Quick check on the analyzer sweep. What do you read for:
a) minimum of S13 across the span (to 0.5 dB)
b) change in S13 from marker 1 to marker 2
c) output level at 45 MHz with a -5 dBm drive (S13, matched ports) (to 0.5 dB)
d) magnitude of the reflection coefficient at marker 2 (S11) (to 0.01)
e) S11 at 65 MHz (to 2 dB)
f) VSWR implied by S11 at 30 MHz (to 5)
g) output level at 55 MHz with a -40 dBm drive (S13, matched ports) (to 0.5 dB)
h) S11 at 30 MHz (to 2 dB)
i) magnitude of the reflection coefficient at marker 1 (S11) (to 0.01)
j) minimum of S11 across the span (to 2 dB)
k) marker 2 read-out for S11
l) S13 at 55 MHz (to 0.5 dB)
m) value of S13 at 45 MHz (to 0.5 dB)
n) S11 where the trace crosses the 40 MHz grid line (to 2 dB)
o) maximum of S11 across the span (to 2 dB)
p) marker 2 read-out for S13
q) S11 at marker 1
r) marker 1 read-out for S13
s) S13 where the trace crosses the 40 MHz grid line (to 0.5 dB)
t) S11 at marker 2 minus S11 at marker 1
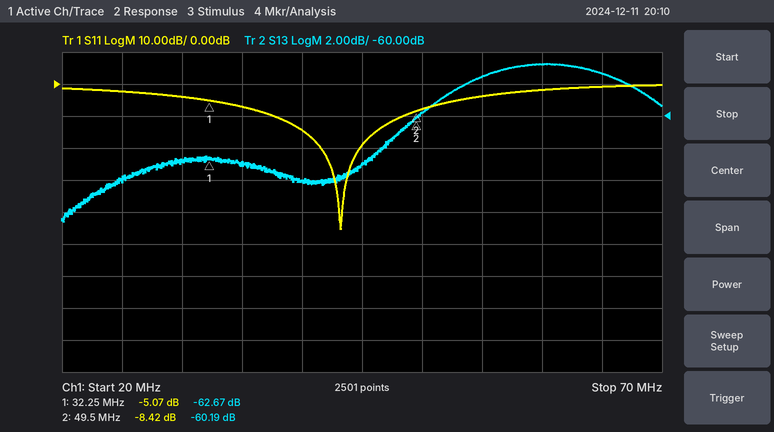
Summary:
-66.5 dB
2.48 dB
-68.0 dBm
0.38
0 dB
5
-97.5 dBm
-4 dB
0.56
-46 dB
-8.42 dB
-57.5 dB
-63.0 dB
-14 dB
0 dB
-60.19 dB
-5.07 dB
-62.67 dB
-64.0 dB
-3.35 dB
